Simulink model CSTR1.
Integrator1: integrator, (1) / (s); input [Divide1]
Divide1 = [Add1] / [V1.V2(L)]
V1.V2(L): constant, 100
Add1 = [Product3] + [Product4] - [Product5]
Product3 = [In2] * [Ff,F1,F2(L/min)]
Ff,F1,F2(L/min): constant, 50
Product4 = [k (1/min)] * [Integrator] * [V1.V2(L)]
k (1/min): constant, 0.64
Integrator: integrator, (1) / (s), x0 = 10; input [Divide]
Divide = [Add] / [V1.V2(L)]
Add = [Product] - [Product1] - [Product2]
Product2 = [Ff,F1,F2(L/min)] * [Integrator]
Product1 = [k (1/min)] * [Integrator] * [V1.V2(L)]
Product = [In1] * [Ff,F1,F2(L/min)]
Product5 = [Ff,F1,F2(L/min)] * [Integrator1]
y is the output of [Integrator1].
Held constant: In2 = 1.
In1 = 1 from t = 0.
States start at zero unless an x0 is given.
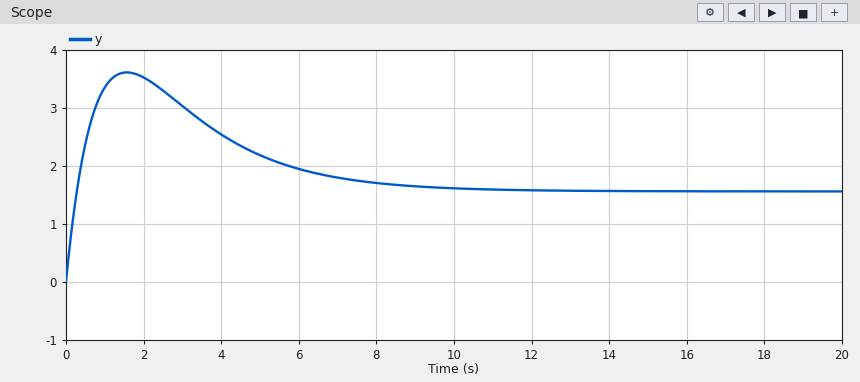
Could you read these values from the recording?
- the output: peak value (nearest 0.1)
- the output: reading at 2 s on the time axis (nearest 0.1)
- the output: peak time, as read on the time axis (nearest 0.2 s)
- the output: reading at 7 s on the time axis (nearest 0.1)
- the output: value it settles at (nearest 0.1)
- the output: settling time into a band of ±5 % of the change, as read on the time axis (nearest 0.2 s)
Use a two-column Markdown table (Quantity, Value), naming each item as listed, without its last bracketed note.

| Quantity | Value |
|---|---|
| the output: peak value | 3.6 |
| the output: reading at 2 s on the time axis | 3.5 |
| the output: peak time, as read on the time axis | 1.6 s |
| the output: reading at 7 s on the time axis | 1.8 |
| the output: value it settles at | 1.6 |
| the output: settling time into a band of ±5 % of the change, as read on the time axis | 9.2 s |
